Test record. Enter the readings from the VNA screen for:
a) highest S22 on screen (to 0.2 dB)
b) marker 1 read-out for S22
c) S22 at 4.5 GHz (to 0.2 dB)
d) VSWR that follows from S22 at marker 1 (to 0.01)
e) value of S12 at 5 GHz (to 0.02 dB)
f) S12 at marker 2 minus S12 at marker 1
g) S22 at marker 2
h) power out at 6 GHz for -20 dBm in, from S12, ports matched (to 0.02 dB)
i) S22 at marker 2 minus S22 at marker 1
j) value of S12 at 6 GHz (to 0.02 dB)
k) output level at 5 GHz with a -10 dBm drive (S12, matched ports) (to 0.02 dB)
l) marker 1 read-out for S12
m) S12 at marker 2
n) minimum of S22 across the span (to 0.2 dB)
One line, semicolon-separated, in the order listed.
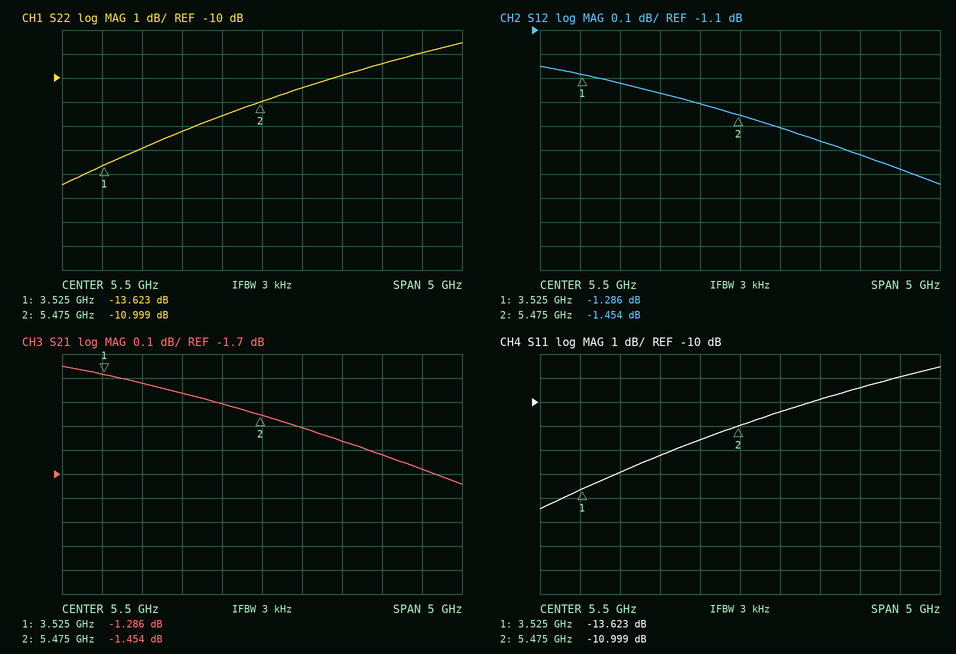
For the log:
-8.6 dB; -13.623 dB; -12.2 dB; 1.53; -1.40 dB; -0.168 dB; -10.999 dB; -21.50 dBm; 2.624 dB; -1.50 dB; -11.40 dBm; -1.286 dB; -1.454 dB; -14.4 dB
